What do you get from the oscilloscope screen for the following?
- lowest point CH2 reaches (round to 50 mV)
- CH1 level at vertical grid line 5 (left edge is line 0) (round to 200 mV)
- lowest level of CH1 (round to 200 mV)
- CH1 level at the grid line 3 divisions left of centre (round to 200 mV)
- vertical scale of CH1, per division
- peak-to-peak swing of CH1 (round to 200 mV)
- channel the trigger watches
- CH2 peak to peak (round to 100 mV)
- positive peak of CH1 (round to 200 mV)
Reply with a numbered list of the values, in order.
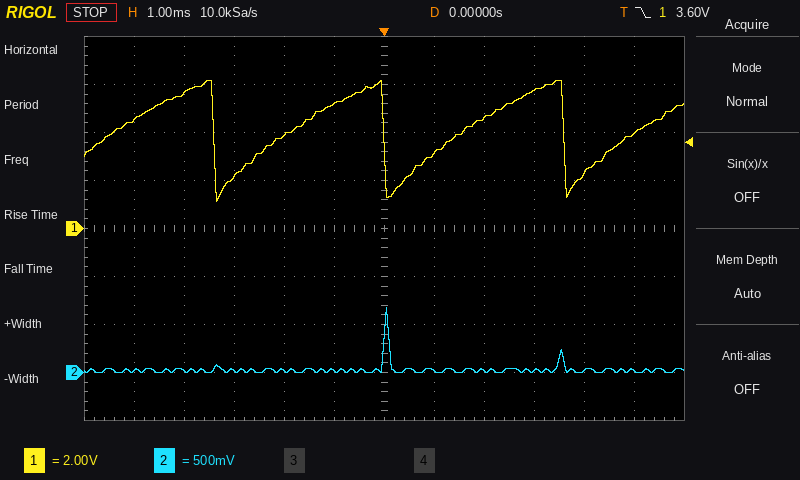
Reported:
1. 0 mV
2. 5.2 V
3. 1.2 V
4. 2.2 V
5. 2 V
6. 5.0 V
7. CH1
8. 700 mV
9. 6.2 V
